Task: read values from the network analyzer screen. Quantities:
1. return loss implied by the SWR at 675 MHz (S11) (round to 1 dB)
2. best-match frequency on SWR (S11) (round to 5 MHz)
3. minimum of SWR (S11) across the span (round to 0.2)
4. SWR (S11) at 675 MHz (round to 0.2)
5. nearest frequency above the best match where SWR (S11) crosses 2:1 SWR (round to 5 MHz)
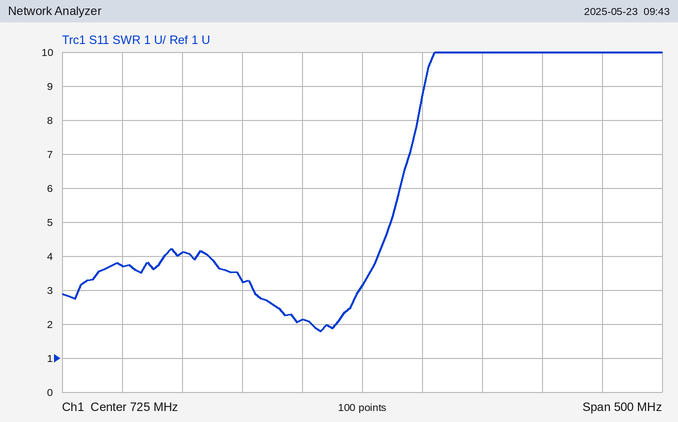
9 dB
690 MHz
1.8
2.2
705 MHz
